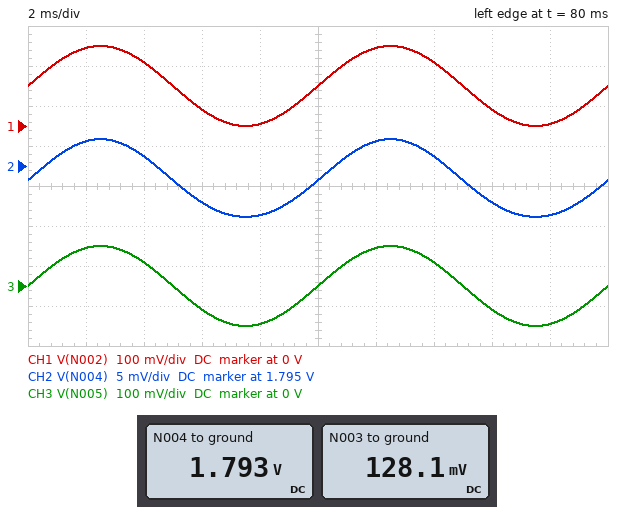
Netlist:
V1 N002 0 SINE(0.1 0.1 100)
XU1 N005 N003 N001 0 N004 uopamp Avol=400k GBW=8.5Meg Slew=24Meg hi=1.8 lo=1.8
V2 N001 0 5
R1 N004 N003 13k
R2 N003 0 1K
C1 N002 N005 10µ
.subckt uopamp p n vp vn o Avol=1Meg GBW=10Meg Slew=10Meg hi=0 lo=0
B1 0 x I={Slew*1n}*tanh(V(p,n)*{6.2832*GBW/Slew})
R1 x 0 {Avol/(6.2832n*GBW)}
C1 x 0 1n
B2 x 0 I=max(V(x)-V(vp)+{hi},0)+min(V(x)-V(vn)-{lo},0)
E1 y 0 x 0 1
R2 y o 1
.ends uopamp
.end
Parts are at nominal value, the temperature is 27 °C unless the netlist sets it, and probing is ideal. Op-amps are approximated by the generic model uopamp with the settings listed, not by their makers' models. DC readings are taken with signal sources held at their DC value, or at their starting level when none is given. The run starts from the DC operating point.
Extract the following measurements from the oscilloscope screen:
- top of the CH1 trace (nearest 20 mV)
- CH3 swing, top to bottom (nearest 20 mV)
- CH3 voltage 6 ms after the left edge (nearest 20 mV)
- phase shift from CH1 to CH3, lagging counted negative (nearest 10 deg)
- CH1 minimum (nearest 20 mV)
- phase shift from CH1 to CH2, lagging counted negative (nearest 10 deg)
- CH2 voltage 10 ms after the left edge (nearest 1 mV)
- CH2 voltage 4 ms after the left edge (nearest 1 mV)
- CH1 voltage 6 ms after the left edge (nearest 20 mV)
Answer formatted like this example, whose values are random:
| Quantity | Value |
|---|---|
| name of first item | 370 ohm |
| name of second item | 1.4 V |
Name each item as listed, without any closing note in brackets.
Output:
| Quantity | Value |
|---|---|
| top of the CH1 trace | 200 mV |
| CH3 swing, top to bottom | 200 mV |
| CH3 voltage 6 ms after the left edge | -60 mV |
| phase shift from CH1 to CH3, lagging counted negative | 0 deg |
| CH1 minimum | 0 V |
| phase shift from CH1 to CH2, lagging counted negative | 0 deg |
| CH2 voltage 10 ms after the left edge | 1.793 V |
| CH2 voltage 4 ms after the left edge | 1.796 V |
| CH1 voltage 6 ms after the left edge | 40 mV |
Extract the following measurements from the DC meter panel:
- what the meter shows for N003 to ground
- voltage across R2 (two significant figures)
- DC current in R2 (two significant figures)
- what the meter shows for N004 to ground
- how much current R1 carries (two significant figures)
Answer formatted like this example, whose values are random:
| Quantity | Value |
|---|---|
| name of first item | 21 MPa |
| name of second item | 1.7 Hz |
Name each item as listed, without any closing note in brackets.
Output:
| Quantity | Value |
|---|---|
| what the meter shows for N003 to ground | 128.1 mV |
| voltage across R2 | 130 mV |
| DC current in R2 | 130 µA |
| what the meter shows for N004 to ground | 1.793 V |
| how much current R1 carries | 130 µA |
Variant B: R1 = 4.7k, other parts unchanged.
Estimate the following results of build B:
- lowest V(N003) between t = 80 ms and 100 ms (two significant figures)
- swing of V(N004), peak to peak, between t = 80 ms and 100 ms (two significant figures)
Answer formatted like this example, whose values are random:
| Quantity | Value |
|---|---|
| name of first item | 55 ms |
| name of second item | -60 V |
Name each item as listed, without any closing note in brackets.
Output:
| Quantity | Value |
|---|---|
| lowest V(N003) between t = 80 ms and 100 ms | 310 mV |
| swing of V(N004), peak to peak, between t = 80 ms and 100 ms | 6.8 mV |
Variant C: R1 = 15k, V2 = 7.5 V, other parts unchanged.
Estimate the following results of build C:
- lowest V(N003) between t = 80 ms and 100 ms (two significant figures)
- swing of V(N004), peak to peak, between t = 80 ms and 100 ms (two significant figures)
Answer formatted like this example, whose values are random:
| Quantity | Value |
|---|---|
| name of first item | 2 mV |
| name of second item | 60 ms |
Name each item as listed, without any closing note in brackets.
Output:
| Quantity | Value |
|---|---|
| lowest V(N003) between t = 80 ms and 100 ms | 110 mV |
| swing of V(N004), peak to peak, between t = 80 ms and 100 ms | 9.9 mV |
